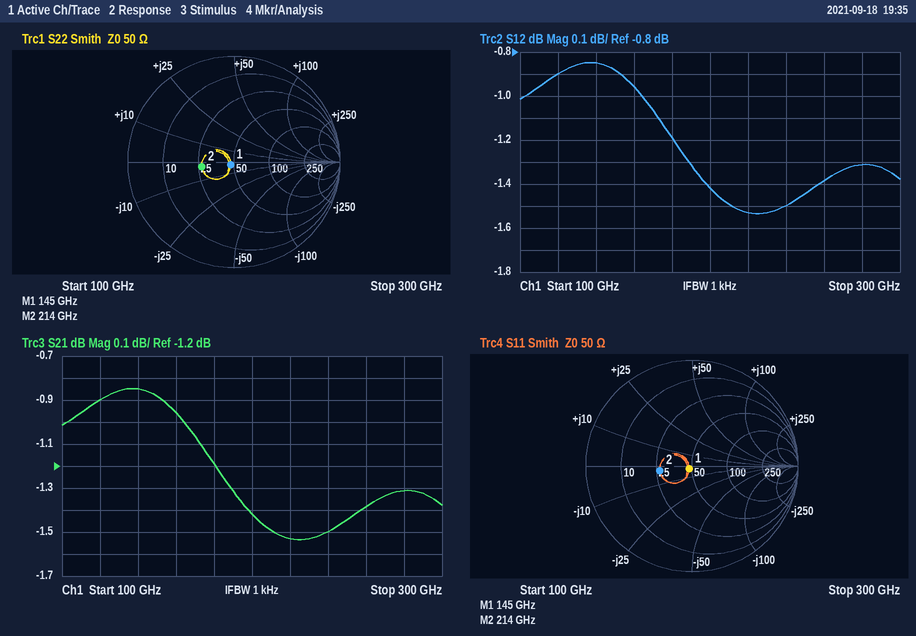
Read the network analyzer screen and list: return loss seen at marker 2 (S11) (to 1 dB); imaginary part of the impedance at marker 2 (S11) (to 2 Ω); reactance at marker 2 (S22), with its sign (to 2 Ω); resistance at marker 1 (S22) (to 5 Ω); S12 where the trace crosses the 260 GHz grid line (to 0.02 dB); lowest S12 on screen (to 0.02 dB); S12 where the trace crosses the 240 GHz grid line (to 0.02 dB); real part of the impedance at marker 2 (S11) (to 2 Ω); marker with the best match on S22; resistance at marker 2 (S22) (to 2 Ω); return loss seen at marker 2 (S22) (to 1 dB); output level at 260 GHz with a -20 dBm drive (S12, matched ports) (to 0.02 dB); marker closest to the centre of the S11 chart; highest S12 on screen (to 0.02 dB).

10 dB
-2 Ω
-2 Ω
45 Ω
-1.38 dB
-1.54 dB
-1.50 dB
26 Ω
marker 1
26 Ω
10 dB
-21.38 dBm
marker 1
-0.84 dB
